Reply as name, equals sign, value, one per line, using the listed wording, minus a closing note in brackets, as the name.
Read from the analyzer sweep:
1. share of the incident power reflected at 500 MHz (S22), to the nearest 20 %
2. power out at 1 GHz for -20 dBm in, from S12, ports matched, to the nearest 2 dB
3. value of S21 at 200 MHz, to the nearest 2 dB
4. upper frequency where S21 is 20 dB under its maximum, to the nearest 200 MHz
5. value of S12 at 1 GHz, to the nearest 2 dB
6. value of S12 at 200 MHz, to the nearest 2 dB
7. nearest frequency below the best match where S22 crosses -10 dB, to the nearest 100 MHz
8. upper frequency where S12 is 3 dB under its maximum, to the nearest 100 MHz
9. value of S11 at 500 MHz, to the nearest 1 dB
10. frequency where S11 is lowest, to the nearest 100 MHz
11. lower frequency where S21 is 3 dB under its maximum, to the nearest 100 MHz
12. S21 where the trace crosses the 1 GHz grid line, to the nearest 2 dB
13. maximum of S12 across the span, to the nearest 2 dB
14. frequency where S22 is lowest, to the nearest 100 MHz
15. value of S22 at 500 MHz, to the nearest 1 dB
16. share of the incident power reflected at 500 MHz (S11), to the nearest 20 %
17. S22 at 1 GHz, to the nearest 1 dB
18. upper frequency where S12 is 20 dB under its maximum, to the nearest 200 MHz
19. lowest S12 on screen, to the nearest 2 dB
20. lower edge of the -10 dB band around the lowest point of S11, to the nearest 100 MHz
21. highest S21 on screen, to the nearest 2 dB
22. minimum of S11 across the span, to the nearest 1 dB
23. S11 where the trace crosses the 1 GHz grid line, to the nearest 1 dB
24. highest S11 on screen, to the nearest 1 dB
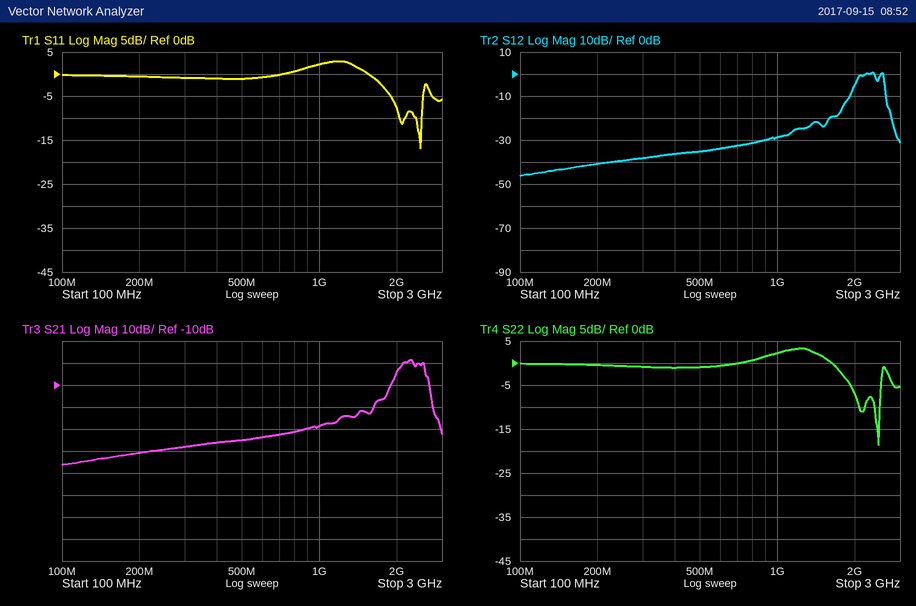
share of the incident power reflected at 500 MHz (S22), to the nearest 20 % = 80 %
power out at 1 GHz for -20 dBm in, from S12, ports matched, to the nearest 2 dB = -48 dBm
value of S21 at 200 MHz, to the nearest 2 dB = -40 dB
upper frequency where S21 is 20 dB under its maximum, to the nearest 200 MHz = 2.8 GHz
value of S12 at 1 GHz, to the nearest 2 dB = -28 dB
value of S12 at 200 MHz, to the nearest 2 dB = -40 dB
nearest frequency below the best match where S22 crosses -10 dB, to the nearest 100 MHz = 2.4 GHz
upper frequency where S12 is 3 dB under its maximum, to the nearest 100 MHz = 2.4 GHz
value of S11 at 500 MHz, to the nearest 1 dB = -1 dB
frequency where S11 is lowest, to the nearest 100 MHz = 2.5 GHz
lower frequency where S21 is 3 dB under its maximum, to the nearest 100 MHz = 2.1 GHz
S21 where the trace crosses the 1 GHz grid line, to the nearest 2 dB = -28 dB
maximum of S12 across the span, to the nearest 2 dB = 0 dB
frequency where S22 is lowest, to the nearest 100 MHz = 2.5 GHz
value of S22 at 500 MHz, to the nearest 1 dB = -1 dB
share of the incident power reflected at 500 MHz (S11), to the nearest 20 % = 80 %
S22 at 1 GHz, to the nearest 1 dB = 2 dB
upper frequency where S12 is 20 dB under its maximum, to the nearest 200 MHz = 2.8 GHz
lowest S12 on screen, to the nearest 2 dB = -46 dB
lower edge of the -10 dB band around the lowest point of S11, to the nearest 100 MHz = 2.4 GHz
highest S21 on screen, to the nearest 2 dB = 2 dB
minimum of S11 across the span, to the nearest 1 dB = -17 dB
S11 where the trace crosses the 1 GHz grid line, to the nearest 1 dB = 2 dB
highest S11 on screen, to the nearest 1 dB = 3 dB
